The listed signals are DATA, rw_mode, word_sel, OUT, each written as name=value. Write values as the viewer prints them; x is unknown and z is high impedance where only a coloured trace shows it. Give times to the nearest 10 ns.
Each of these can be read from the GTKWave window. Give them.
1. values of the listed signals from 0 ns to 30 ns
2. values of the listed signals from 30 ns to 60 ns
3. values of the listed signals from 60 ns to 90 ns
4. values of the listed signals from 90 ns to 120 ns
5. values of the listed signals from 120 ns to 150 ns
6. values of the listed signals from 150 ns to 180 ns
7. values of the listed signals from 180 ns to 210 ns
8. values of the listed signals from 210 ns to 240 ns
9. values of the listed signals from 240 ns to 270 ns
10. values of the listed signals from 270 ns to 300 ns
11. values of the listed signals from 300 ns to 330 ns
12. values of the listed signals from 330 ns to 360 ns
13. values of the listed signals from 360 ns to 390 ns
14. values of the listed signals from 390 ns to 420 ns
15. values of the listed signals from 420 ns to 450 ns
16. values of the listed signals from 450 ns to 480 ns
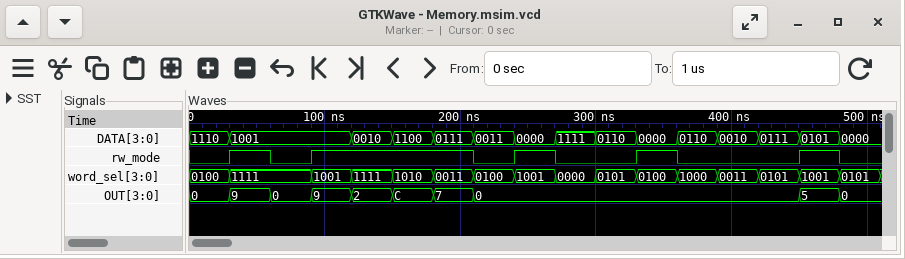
DATA=1110, rw_mode=0, word_sel=0100, OUT=0
DATA=1001, rw_mode=1, word_sel=1111, OUT=9
DATA=1001, rw_mode=0, word_sel=1111, OUT=0
DATA=1001, rw_mode=1, word_sel=1001, OUT=9
DATA=0010, rw_mode=1, word_sel=1111, OUT=2
DATA=1100, rw_mode=1, word_sel=1010, OUT=C
DATA=0111, rw_mode=1, word_sel=0011, OUT=7
DATA=0011, rw_mode=0, word_sel=0100, OUT=0
DATA=0000, rw_mode=1, word_sel=1001, OUT=0
DATA=1111, rw_mode=0, word_sel=0000, OUT=0
DATA=0110, rw_mode=0, word_sel=0101, OUT=0
DATA=0000, rw_mode=1, word_sel=0100, OUT=0
DATA=0110, rw_mode=0, word_sel=1000, OUT=0
DATA=0010, rw_mode=0, word_sel=0011, OUT=0
DATA=0111, rw_mode=0, word_sel=0101, OUT=0
DATA=0101, rw_mode=1, word_sel=1001, OUT=5
